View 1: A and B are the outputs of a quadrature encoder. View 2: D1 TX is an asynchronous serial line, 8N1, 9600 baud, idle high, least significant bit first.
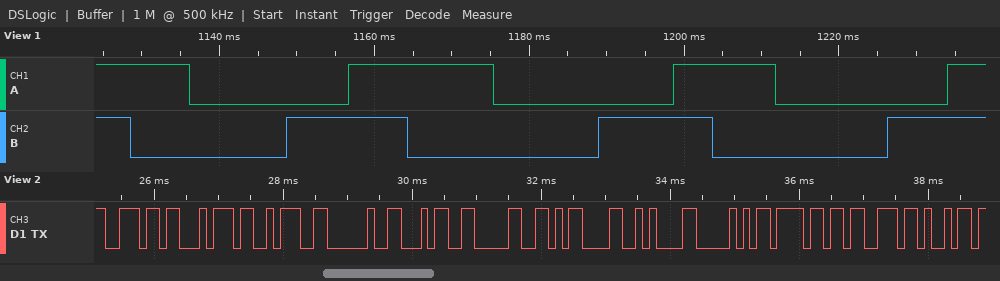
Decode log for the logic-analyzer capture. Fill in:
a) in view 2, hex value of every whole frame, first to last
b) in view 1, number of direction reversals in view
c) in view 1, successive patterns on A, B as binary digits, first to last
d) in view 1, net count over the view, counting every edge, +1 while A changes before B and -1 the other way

6E 74 3A 20 34 30 0D 0A 50 6F 73 69
0
11 10 00 01 11 10 00 01 11 10 00 01 11
-12
